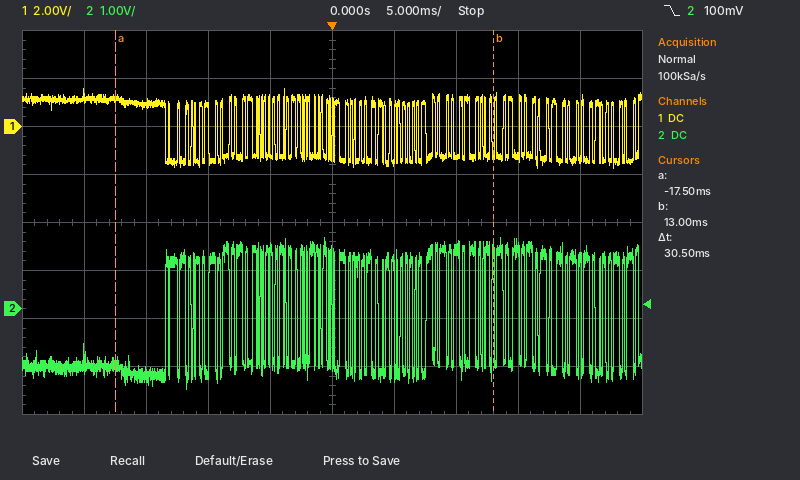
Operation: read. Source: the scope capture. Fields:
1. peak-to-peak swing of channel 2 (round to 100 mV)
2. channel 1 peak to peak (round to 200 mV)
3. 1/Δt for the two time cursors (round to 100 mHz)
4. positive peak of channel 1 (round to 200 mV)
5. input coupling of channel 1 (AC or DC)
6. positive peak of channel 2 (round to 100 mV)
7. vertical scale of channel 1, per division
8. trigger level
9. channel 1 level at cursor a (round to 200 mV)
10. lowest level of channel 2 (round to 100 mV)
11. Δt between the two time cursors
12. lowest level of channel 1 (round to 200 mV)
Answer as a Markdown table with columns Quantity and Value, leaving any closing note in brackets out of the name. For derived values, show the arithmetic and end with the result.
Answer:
| Quantity | Value |
|---|---|
| peak-to-peak swing of channel 2 | 1.5 V − (-1.7 V) = 3.2 V |
| channel 1 peak to peak | 1.6 V − (-1.8 V) = 3.4 V |
| 1/Δt for the two time cursors | 1 / 30.5 ms ≈ 32.8 Hz |
| positive peak of channel 1 | 1.6 V |
| input coupling of channel 1 | DC |
| positive peak of channel 2 | 1.5 V |
| vertical scale of channel 1, per division | 2 V |
| trigger level | 100 mV |
| channel 1 level at cursor a | 1.2 V |
| lowest level of channel 2 | -1.7 V |
| Δt between the two time cursors | 30.5 ms |
| lowest level of channel 1 | -1.8 V |
